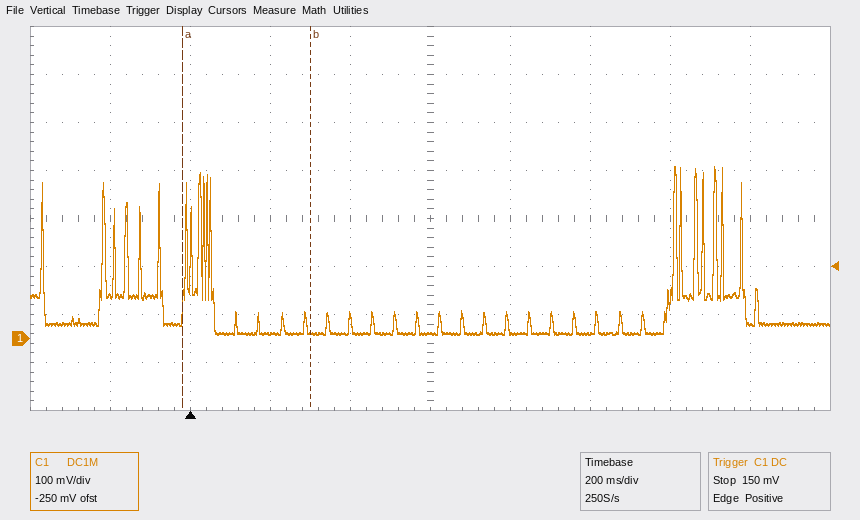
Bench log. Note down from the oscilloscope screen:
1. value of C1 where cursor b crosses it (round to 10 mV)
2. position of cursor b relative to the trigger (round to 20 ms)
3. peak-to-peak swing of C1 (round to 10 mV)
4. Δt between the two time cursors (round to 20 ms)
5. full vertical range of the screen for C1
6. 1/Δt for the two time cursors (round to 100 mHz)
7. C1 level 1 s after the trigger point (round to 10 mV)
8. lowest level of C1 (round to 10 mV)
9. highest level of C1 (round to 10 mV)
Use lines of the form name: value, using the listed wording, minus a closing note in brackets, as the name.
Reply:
value of C1 where cursor b crosses it: 20 mV
position of cursor b relative to the trigger: +300 ms
peak-to-peak swing of C1: 350 mV
Δt between the two time cursors: 320 ms
full vertical range of the screen for C1: 800 mV
1/Δt for the two time cursors: 3.1 Hz
C1 level 1 s after the trigger point: 10 mV
lowest level of C1: 10 mV
highest level of C1: 360 mV
